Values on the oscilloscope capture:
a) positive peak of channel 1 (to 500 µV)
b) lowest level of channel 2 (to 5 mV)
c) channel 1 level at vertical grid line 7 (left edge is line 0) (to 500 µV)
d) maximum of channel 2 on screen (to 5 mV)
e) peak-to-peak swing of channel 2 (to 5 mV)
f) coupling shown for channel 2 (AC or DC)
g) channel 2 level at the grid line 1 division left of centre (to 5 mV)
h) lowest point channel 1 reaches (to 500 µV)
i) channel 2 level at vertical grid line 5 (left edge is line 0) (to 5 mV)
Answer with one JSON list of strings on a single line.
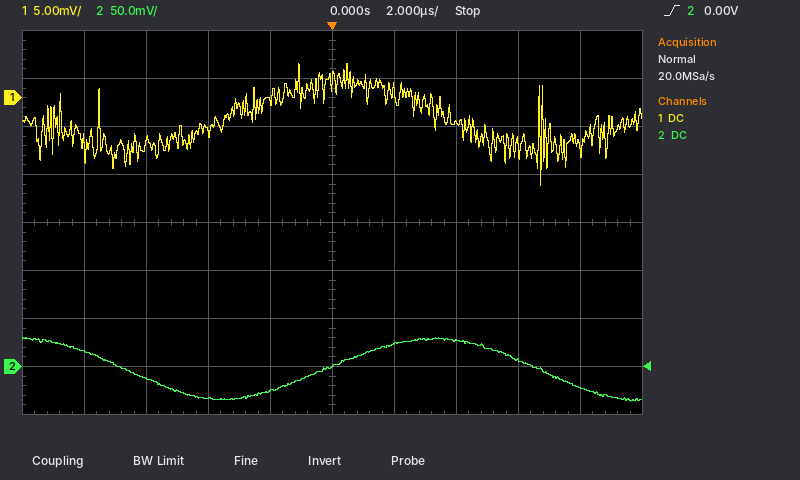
["3.5 mV", "-35 mV", "-2.5 mV", "30 mV", "65 mV", "DC", "-25 mV", "-9.0 mV", "0 mV"]
